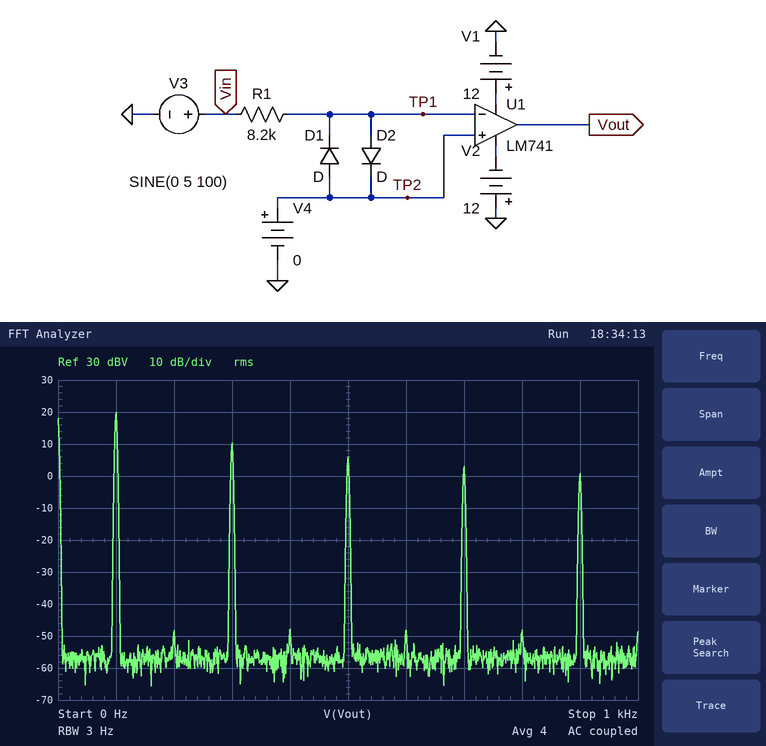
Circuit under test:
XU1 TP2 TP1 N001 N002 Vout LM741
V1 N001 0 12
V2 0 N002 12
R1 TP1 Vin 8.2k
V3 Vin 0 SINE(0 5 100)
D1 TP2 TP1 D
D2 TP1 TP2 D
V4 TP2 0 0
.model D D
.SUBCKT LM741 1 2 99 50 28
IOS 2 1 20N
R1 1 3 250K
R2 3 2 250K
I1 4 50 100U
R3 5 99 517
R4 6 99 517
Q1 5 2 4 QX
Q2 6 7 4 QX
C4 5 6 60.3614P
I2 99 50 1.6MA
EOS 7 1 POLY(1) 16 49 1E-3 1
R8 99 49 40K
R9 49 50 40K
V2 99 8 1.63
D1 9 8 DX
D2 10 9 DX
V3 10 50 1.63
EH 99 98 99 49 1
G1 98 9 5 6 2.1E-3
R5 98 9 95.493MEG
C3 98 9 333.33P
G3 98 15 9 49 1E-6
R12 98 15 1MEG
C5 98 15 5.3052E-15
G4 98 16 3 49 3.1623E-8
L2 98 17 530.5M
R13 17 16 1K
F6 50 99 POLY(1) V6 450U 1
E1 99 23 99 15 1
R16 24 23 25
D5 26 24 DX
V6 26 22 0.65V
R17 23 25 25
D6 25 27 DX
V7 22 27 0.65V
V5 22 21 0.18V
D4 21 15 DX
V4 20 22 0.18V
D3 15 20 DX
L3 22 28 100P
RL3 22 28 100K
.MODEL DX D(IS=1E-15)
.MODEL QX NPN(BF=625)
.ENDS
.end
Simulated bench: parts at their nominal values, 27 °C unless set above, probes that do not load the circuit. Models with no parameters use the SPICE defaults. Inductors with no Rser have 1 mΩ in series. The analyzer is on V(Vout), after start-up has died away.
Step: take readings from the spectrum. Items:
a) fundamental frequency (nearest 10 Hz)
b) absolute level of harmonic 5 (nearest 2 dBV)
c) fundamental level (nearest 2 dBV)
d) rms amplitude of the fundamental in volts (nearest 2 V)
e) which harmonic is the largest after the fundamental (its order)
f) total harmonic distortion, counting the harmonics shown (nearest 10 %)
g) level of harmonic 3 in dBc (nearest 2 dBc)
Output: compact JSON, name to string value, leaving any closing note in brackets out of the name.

{"fundamental frequency": "100 Hz", "absolute level of harmonic 5": "6 dBV", "fundamental level": "20 dBV", "rms amplitude of the fundamental in volts": "10 V", "which harmonic is the largest after the fundamental": "3", "total harmonic distortion, counting the harmonics shown": "40 %", "level of harmonic 3 in dBc": "-10 dBc"}
